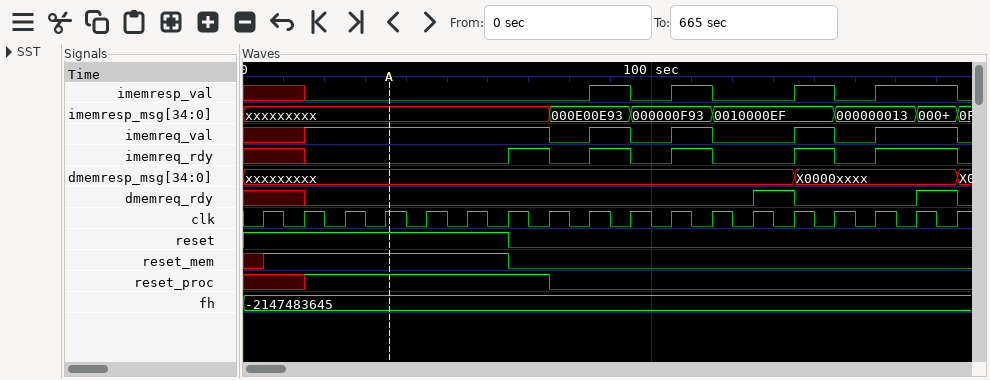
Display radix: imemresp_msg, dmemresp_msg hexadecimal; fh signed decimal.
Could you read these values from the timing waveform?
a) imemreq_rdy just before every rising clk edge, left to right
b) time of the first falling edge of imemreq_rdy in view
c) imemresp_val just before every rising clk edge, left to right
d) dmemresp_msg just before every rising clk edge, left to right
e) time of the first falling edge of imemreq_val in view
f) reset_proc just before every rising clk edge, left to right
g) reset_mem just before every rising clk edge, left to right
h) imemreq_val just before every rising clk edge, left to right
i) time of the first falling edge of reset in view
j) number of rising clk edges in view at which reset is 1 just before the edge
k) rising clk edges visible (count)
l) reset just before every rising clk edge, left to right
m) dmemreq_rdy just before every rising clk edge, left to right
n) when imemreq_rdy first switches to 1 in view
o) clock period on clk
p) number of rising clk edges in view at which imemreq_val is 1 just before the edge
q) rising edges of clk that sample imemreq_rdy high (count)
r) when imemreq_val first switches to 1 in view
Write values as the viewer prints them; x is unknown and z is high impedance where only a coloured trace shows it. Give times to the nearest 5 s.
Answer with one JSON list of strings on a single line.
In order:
["x x 0 0 0 0 0 1 0 1 0 1 0 0 1 0 1 1", "75 s", "x x 0 0 0 0 0 0 0 1 0 1 0 0 1 0 1 1", "xxxxxxxxx, xxxxxxxxx, xxxxxxxxx, xxxxxxxxx, xxxxxxxxx, xxxxxxxxx, xxxxxxxxx, xxxxxxxxx, xxxxxxxxx, xxxxxxxxx, xxxxxxxxx, xxxxxxxxx, xxxxxxxxx, xxxxxxxxx, X0000xxxx, X0000xxxx, X0000xxxx, X0000xxxx", "75 s", "x x 1 1 1 1 1 1 0 0 0 0 0 0 0 0 0 0", "x 1 1 1 1 1 1 0 0 0 0 0 0 0 0 0 0 0", "x x 1 1 1 1 1 1 0 1 0 1 0 0 1 0 1 1", "65 s", "7", "18", "1 1 1 1 1 1 1 0 0 0 0 0 0 0 0 0 0 0", "x x 0 0 0 0 0 0 0 0 0 0 0 1 0 0 0 1", "65 s", "10 s", "11", "6", "15 s"]
